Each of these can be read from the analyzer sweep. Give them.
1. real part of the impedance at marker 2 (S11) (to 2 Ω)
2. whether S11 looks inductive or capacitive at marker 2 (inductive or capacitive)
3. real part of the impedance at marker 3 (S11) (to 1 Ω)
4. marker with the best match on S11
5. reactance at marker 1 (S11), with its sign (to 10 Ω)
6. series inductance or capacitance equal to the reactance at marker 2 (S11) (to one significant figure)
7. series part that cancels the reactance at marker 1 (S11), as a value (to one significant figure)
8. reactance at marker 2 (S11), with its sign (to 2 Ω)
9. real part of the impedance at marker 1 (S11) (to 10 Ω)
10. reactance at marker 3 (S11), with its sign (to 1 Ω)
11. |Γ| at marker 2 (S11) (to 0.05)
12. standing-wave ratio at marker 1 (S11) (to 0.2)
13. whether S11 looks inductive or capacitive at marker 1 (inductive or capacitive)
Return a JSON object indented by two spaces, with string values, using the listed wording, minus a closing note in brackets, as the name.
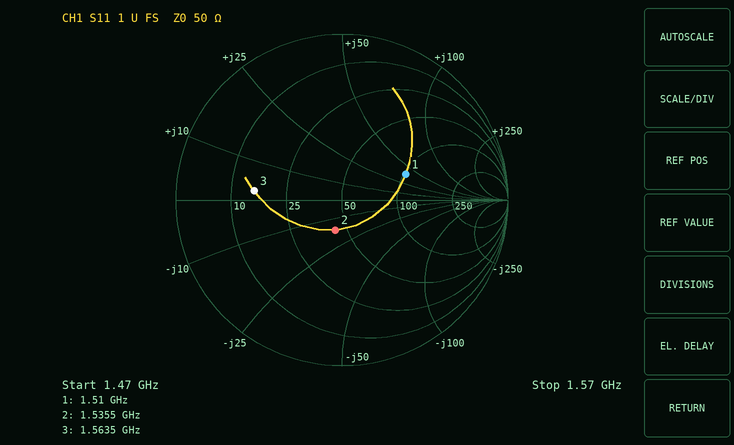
{
  "real part of the impedance at marker 2 (S11)": "44 Ω",
  "whether S11 looks inductive or capacitive at marker 2": "capacitive",
  "real part of the impedance at marker 3 (S11)": "15 Ω",
  "marker with the best match on S11": "marker 2",
  "reactance at marker 1 (S11), with its sign": "+40 Ω",
  "series inductance or capacitance equal to the reactance at marker 2 (S11)": "6 pF",
  "series part that cancels the reactance at marker 1 (S11), as a value": "3 pF",
  "reactance at marker 2 (S11), with its sign": "-16 Ω",
  "real part of the impedance at marker 1 (S11)": "100 Ω",
  "reactance at marker 3 (S11), with its sign": "+2 Ω",
  "|Γ| at marker 2 (S11)": "0.20",
  "standing-wave ratio at marker 1 (S11)": "2.4",
  "whether S11 looks inductive or capacitive at marker 1": "inductive"
}
